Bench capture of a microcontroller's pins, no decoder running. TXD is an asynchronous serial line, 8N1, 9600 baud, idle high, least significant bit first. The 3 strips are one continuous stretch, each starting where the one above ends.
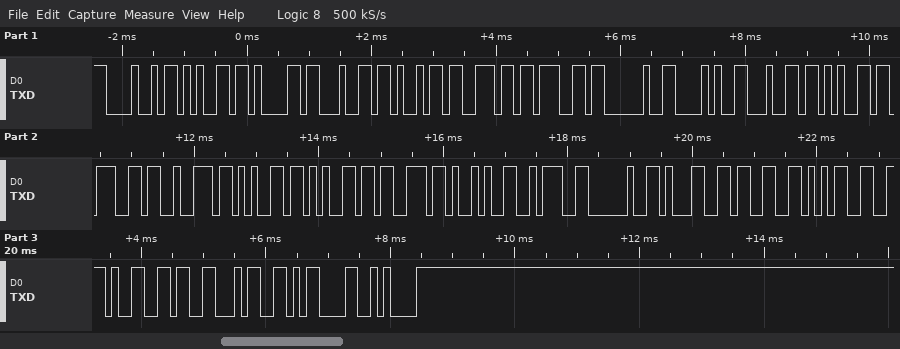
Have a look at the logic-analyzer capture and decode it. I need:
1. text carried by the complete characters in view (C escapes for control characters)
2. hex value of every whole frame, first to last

"Heading (degrees): 135.64\r\n"
48 65 61 64 69 6E 67 20 28 64 65 67 72 65 65 73 29 3A 20 31 33 35 2E 36 34 0D 0A
